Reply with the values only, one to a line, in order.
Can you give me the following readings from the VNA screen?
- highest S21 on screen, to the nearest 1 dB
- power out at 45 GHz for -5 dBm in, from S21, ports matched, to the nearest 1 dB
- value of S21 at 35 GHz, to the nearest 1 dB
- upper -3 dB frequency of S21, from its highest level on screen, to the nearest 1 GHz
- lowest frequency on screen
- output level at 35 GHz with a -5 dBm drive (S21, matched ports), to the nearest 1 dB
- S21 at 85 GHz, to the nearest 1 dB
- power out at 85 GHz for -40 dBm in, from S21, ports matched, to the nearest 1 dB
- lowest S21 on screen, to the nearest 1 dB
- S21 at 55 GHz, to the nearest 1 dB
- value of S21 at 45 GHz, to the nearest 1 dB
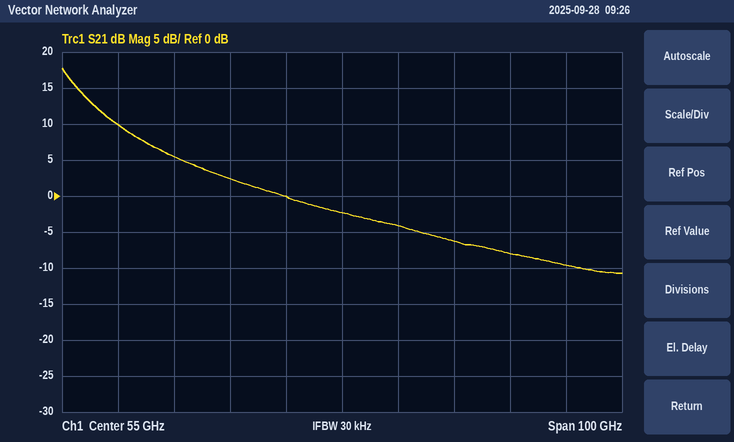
18 dB
-5 dBm
2 dB
8 GHz
5 GHz
-3 dBm
-8 dB
-48 dBm
-11 dB
-2 dB
0 dB
